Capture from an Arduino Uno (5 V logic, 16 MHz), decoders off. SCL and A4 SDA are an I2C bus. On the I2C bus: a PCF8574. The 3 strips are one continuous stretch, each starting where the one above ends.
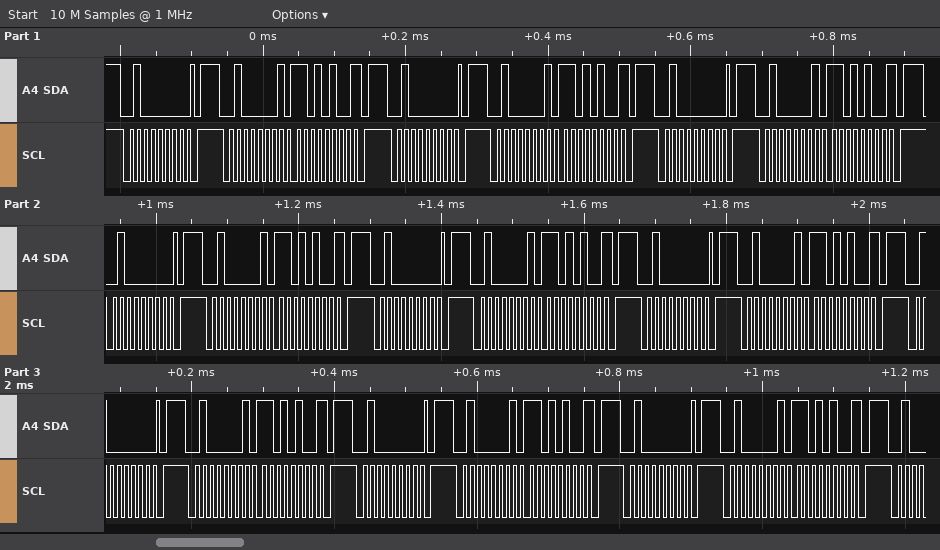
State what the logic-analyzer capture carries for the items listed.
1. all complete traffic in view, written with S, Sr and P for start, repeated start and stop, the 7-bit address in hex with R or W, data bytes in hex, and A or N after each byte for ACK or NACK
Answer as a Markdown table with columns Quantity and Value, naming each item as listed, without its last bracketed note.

| Quantity | Value |
|---|---|
| all complete traffic in view, written with S, Sr and P for start, repeated start and stop, the 7-bit address in hex with R or W, data bytes in hex, and A or N after each byte for ACK or NACK | S 20W A P S 20R A D4 N P S 20W A P S 20R A D4 N P S 20W A P S 20R A D4 N P S 20W A P S 20R A D4 N P S 20W A P S 20R A D4 N P S 20W A P S 20R A D4 N P S 20W A P S 20R A D4 N P S 20W A P S 20R A D4 N P S 20W A P S 20R A D4 N P |
